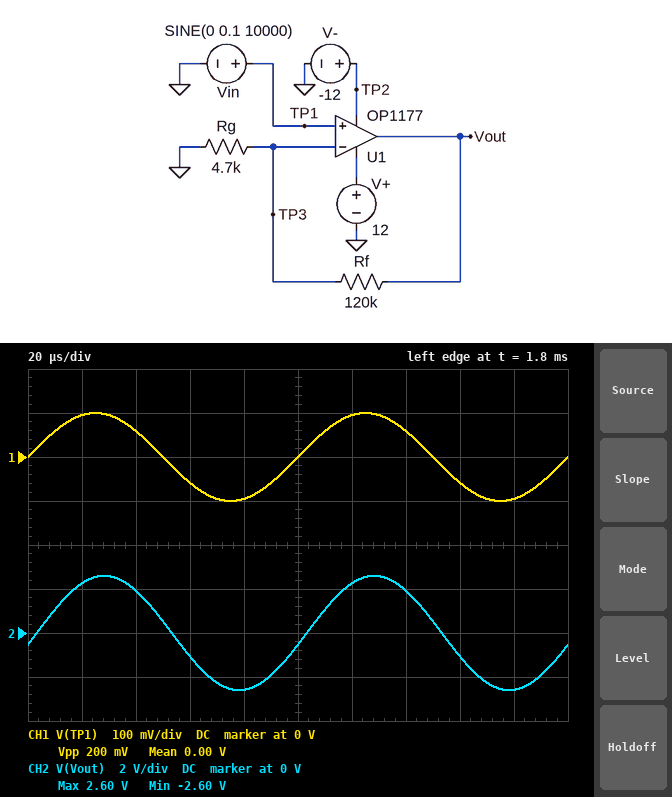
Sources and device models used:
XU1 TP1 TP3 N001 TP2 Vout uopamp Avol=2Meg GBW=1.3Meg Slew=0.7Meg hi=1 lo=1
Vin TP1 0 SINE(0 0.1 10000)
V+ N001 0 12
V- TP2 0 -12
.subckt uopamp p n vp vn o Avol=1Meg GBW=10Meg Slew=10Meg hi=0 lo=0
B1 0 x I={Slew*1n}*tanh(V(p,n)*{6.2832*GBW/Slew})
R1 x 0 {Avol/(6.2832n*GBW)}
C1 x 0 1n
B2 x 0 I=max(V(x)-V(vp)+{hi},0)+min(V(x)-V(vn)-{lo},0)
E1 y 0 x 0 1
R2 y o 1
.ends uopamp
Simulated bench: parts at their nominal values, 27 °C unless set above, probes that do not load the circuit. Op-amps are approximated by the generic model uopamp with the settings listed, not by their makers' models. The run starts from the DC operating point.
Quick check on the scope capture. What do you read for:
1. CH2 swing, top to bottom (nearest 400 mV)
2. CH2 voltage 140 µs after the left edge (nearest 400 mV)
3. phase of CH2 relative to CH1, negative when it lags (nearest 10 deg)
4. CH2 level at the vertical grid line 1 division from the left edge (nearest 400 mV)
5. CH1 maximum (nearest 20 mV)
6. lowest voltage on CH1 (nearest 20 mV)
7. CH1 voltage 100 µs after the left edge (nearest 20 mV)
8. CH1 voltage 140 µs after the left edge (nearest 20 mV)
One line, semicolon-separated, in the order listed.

5.2 V; 2.0 V; -10 deg; 2.4 V; 100 mV; -100 mV; 0 V; 60 mV
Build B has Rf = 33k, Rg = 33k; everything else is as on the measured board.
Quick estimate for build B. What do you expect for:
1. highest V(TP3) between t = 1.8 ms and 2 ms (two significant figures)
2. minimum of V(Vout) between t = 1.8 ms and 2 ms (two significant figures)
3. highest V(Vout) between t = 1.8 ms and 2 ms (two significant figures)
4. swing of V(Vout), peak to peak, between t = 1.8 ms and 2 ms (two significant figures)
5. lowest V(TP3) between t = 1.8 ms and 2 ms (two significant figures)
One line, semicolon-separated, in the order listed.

100 mV; -200 mV; 200 mV; 400 mV; -100 mV
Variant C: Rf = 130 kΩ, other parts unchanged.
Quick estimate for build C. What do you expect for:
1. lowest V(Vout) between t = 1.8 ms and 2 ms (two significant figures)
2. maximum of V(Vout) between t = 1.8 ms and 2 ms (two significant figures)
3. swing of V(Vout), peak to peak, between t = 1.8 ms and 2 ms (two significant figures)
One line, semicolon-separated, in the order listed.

-2.8 V; 2.8 V; 5.6 V
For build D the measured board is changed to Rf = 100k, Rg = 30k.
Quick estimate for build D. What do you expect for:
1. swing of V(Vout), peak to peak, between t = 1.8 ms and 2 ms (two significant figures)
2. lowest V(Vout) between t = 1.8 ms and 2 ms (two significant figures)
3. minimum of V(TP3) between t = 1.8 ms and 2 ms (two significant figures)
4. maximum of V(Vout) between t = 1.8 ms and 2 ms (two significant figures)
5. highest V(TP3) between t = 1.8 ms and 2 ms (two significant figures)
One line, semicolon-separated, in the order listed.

870 mV; -430 mV; -100 mV; 430 mV; 100 mV
